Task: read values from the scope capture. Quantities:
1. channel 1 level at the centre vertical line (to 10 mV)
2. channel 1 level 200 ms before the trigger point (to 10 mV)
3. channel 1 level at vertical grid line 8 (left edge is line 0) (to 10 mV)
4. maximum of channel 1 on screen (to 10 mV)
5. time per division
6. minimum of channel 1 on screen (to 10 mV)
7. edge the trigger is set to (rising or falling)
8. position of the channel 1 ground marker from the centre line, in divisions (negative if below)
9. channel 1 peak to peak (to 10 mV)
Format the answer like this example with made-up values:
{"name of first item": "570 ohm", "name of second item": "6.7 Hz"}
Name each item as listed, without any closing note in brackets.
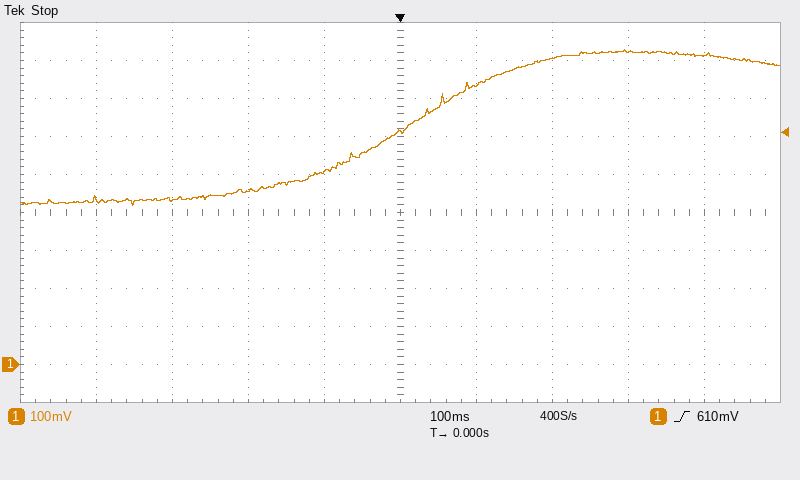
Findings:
{"channel 1 level at the centre vertical line": "610 mV", "channel 1 level 200 ms before the trigger point": "460 mV", "channel 1 level at vertical grid line 8 (left edge is line 0)": "820 mV", "maximum of channel 1 on screen": "830 mV", "time per division": "100 ms", "minimum of channel 1 on screen": "420 mV", "edge the trigger is set to": "rising", "position of the channel 1 ground marker from the centre line, in divisions": "-4.0 div", "channel 1 peak to peak": "410 mV"}
